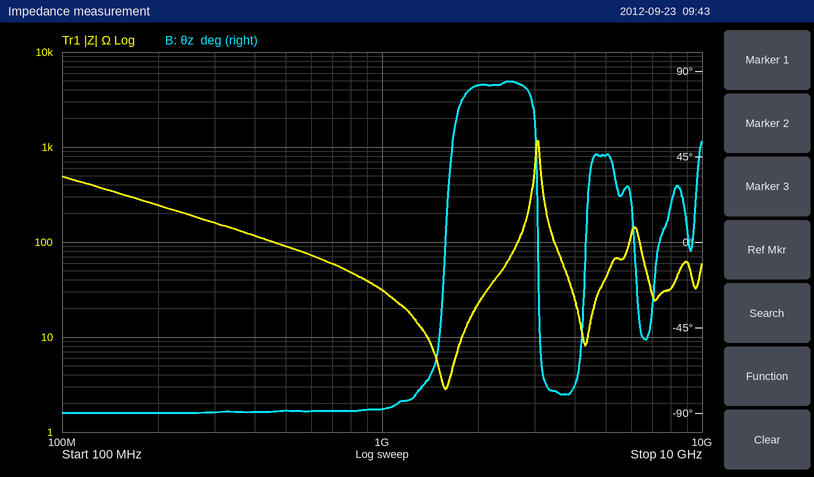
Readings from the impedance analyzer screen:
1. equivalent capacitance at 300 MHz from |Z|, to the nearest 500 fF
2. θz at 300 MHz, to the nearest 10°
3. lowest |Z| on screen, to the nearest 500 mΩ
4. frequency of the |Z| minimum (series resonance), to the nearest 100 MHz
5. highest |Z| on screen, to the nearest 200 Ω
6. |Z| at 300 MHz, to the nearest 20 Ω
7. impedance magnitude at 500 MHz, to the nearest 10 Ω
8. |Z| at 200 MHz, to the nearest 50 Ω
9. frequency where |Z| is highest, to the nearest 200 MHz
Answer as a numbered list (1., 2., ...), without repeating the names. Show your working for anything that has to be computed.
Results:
1. C = 1/(2π × 300 MHz × 160 Ω) ≈ 3.32 pF, so 3.5 pF to the nearest 500 fF
2. -90°
3. 3.0 Ω
4. 1.6 GHz
5. 1.2 kΩ
6. 160 Ω
7. 90 Ω
8. 250 Ω
9. 3.0 GHz
